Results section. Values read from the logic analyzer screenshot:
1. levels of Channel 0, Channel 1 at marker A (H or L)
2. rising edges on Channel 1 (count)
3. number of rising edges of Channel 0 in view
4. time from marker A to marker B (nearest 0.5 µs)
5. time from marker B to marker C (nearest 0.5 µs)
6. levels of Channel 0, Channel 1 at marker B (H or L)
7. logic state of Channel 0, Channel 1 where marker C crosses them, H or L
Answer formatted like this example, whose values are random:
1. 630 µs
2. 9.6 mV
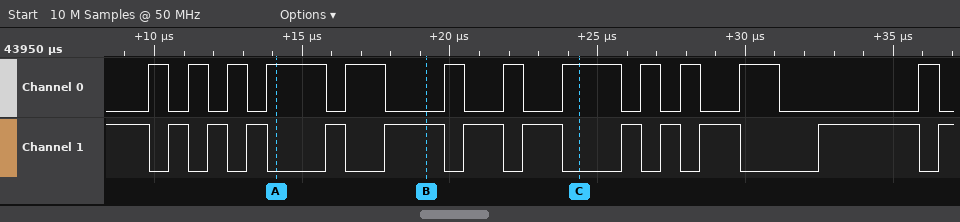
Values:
1. Channel 0=H, Channel 1=L
2. 12
3. 12
4. 5 µs
5. 5 µs
6. Channel 0=L, Channel 1=H
7. Channel 0=H, Channel 1=L
